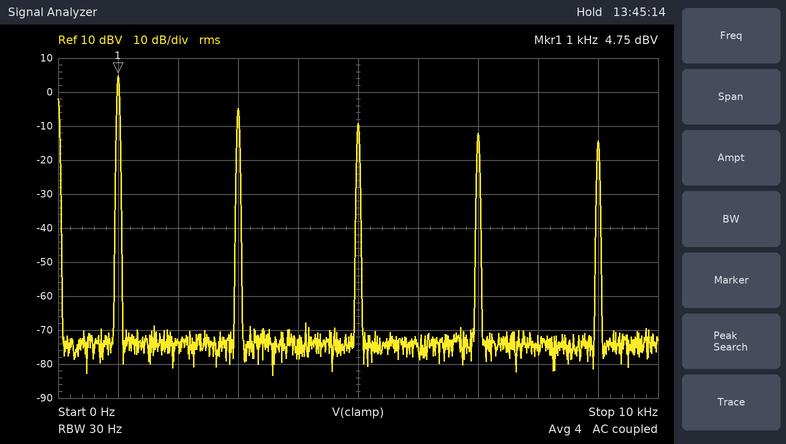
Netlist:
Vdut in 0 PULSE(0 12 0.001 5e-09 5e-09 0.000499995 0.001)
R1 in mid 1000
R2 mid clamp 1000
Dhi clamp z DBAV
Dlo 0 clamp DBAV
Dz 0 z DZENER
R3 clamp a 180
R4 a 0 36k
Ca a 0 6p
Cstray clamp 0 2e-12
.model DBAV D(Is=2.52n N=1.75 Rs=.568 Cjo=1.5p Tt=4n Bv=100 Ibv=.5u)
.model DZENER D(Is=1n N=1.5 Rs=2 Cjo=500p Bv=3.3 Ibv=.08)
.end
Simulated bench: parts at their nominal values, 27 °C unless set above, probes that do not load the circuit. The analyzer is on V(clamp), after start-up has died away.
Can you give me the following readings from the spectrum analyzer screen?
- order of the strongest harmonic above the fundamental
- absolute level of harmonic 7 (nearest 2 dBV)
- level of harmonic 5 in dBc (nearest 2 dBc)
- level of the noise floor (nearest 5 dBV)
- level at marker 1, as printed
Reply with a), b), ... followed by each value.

a) 3
b) -12 dBV
c) -14 dBc
d) -75 dBV
e) 4.75 dBV
